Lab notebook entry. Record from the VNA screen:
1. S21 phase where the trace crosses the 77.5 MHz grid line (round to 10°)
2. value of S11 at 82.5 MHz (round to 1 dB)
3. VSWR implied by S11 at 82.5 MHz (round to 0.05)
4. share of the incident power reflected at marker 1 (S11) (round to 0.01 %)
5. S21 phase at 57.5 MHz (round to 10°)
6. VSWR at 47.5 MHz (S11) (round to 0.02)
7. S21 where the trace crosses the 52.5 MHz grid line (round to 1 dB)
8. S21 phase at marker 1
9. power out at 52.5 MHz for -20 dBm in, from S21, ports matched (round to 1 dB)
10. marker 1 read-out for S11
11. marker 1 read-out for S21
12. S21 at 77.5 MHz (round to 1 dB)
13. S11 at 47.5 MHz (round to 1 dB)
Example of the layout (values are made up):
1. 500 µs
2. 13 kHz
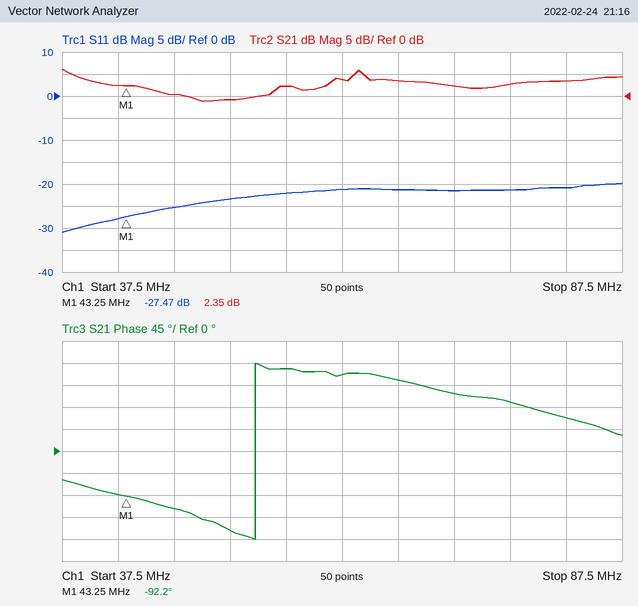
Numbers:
1. 100°
2. -21 dB
3. 1.20
4. 0.18 %
5. 170°
6. 1.12
7. -1 dB
8. -92.2°
9. -21 dBm
10. -27.47 dB
11. 2.35 dB
12. 3 dB
13. -25 dB
